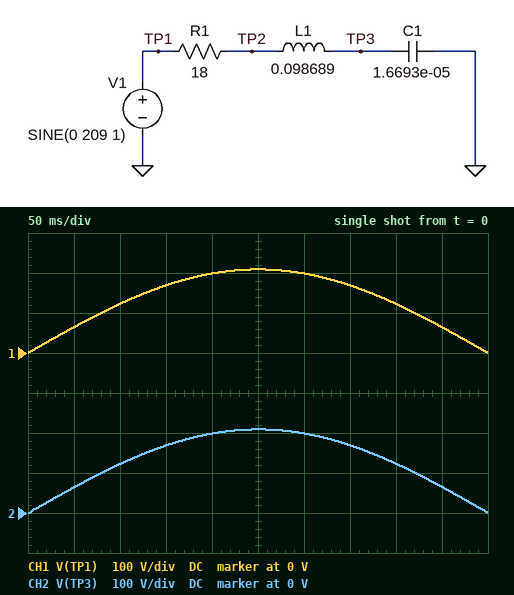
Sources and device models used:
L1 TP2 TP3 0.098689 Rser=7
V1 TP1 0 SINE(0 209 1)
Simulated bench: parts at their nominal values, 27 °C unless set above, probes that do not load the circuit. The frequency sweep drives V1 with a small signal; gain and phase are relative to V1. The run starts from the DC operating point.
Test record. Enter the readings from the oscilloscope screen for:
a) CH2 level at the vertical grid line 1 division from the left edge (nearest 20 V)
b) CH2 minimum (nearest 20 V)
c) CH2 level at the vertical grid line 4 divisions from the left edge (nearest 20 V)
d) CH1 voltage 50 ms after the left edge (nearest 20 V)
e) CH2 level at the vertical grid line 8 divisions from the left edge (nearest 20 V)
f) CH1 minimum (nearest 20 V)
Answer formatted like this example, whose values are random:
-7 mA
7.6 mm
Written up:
60 V
0 V
200 V
60 V
120 V
0 V
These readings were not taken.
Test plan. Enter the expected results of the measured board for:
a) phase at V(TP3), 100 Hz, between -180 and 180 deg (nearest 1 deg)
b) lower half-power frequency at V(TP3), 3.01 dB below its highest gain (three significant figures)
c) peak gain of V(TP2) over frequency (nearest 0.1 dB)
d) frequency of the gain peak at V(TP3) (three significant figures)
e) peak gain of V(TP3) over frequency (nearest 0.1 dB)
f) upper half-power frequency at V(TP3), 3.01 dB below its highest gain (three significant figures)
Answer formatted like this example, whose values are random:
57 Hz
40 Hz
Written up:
-37 deg
98.1 Hz
0 dB
121 Hz
9.9 dB
140 Hz
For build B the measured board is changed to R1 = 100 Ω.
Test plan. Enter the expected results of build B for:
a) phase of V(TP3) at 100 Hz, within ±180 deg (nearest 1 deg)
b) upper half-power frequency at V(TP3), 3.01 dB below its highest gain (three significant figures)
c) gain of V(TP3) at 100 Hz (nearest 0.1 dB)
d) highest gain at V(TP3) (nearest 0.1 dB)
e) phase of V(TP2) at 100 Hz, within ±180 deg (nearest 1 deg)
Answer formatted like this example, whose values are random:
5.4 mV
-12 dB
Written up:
-73 deg
126 Hz
-1.4 dB
0 dB
-61 deg
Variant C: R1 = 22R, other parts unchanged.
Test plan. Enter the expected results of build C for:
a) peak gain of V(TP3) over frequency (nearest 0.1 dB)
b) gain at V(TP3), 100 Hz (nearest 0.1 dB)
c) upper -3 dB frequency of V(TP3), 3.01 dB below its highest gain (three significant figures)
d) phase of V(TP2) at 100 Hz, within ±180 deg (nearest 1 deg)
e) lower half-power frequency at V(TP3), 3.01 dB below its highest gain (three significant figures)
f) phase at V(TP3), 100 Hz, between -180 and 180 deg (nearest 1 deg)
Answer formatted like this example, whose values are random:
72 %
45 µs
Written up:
8.6 dB
6.7 dB
141 Hz
-29 deg
92.7 Hz
-41 deg
